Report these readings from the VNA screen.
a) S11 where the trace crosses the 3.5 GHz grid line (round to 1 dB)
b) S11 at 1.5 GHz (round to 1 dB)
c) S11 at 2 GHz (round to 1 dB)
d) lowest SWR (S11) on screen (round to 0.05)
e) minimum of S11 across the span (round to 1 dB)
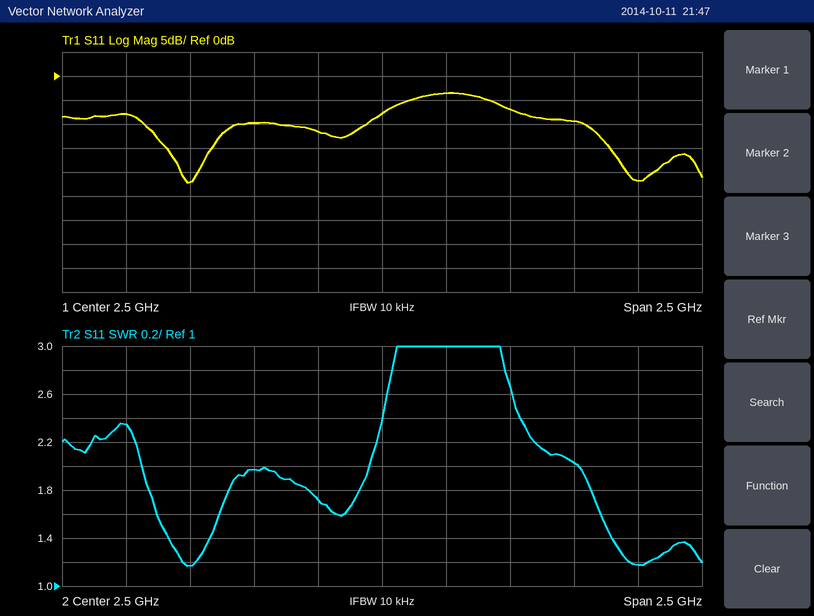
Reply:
-22 dB
-8 dB
-10 dB
1.15
-22 dB
